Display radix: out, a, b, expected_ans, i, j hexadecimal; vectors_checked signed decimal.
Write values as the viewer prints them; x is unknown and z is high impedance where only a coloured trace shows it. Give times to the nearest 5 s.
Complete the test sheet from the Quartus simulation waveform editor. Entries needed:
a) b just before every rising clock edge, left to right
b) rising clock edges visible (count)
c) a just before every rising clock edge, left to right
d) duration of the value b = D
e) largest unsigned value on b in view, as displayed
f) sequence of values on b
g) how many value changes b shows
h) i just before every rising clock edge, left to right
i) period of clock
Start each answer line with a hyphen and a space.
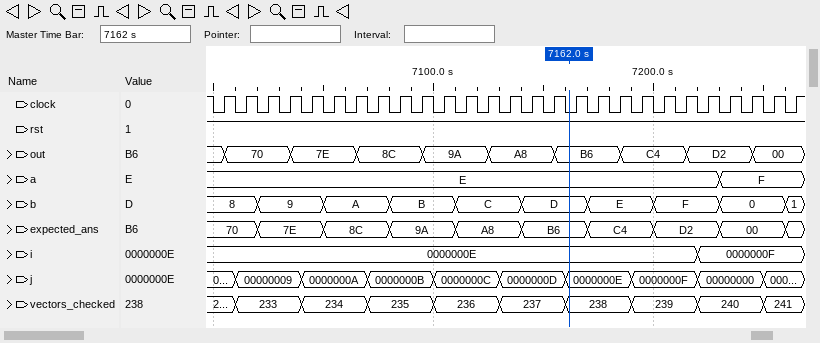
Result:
- 8, 8, 9, 9, 9, A, A, A, B, B, B, C, C, C, D, D, D, E, E, E, F, F, F, 0, 0, 0, 1
- 27
- E, E, E, E, E, E, E, E, E, E, E, E, E, E, E, E, E, E, E, E, E, E, E, F, F, F, F
- 30 s
- F
- 8, 9, A, B, C, D, E, F, 0, 1
- 9
- 0000000E, 0000000E, 0000000E, 0000000E, 0000000E, 0000000E, 0000000E, 0000000E, 0000000E, 0000000E, 0000000E, 0000000E, 0000000E, 0000000E, 0000000E, 0000000E, 0000000E, 0000000E, 0000000E, 0000000E, 0000000E, 0000000E, 0000000F, 0000000F, 0000000F, 0000000F, 0000000F
- 10 s
